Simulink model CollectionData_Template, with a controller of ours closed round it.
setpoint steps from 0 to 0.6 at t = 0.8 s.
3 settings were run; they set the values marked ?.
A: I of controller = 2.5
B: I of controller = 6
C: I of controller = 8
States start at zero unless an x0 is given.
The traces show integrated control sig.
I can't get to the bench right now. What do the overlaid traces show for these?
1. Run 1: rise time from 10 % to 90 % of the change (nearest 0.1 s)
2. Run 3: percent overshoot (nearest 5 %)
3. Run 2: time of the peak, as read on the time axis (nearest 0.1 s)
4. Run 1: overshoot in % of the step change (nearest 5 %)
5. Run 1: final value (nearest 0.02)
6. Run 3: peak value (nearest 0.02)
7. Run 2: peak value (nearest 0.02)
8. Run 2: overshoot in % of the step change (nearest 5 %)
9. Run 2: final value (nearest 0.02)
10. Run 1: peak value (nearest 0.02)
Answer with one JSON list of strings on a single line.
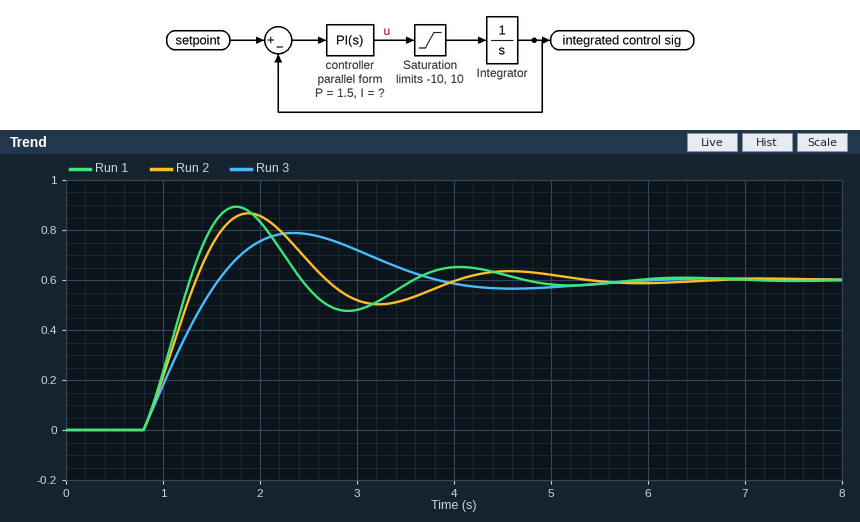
["0.4 s", "30 %", "1.9 s", "50 %", "0.60", "0.78", "0.86", "45 %", "0.60", "0.90"]
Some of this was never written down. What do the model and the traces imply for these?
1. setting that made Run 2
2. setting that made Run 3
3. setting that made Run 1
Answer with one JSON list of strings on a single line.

["B", "A", "C"]
